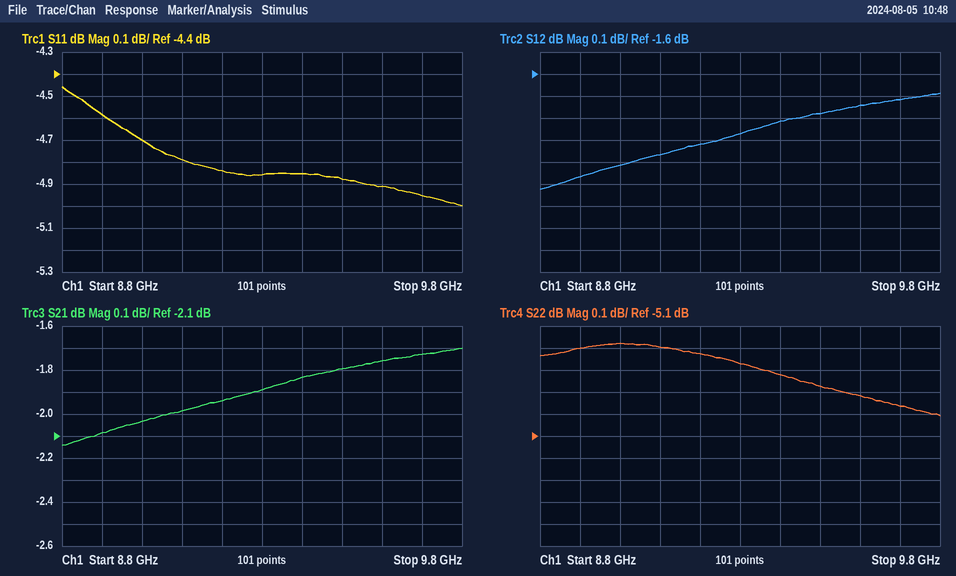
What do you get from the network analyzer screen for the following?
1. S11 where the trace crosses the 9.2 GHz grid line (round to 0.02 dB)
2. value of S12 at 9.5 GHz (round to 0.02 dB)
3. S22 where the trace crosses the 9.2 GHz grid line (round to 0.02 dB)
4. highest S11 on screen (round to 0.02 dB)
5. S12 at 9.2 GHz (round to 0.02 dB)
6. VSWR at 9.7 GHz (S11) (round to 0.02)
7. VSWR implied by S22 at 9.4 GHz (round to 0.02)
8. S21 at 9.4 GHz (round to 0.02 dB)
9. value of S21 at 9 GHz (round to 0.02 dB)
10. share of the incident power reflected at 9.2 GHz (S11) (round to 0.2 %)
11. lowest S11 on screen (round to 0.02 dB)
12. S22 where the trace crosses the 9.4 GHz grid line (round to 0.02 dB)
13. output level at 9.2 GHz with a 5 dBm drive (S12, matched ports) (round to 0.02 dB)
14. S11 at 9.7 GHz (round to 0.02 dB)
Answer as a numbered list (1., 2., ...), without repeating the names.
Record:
1. -4.84 dB
2. -1.78 dB
3. -4.72 dB
4. -4.46 dB
5. -1.92 dB
6. 3.60
7. 3.70
8. -1.84 dB
9. -2.04 dB
10. 32.8 %
11. -5.00 dB
12. -4.82 dB
13. 3.08 dBm
14. -4.96 dB
